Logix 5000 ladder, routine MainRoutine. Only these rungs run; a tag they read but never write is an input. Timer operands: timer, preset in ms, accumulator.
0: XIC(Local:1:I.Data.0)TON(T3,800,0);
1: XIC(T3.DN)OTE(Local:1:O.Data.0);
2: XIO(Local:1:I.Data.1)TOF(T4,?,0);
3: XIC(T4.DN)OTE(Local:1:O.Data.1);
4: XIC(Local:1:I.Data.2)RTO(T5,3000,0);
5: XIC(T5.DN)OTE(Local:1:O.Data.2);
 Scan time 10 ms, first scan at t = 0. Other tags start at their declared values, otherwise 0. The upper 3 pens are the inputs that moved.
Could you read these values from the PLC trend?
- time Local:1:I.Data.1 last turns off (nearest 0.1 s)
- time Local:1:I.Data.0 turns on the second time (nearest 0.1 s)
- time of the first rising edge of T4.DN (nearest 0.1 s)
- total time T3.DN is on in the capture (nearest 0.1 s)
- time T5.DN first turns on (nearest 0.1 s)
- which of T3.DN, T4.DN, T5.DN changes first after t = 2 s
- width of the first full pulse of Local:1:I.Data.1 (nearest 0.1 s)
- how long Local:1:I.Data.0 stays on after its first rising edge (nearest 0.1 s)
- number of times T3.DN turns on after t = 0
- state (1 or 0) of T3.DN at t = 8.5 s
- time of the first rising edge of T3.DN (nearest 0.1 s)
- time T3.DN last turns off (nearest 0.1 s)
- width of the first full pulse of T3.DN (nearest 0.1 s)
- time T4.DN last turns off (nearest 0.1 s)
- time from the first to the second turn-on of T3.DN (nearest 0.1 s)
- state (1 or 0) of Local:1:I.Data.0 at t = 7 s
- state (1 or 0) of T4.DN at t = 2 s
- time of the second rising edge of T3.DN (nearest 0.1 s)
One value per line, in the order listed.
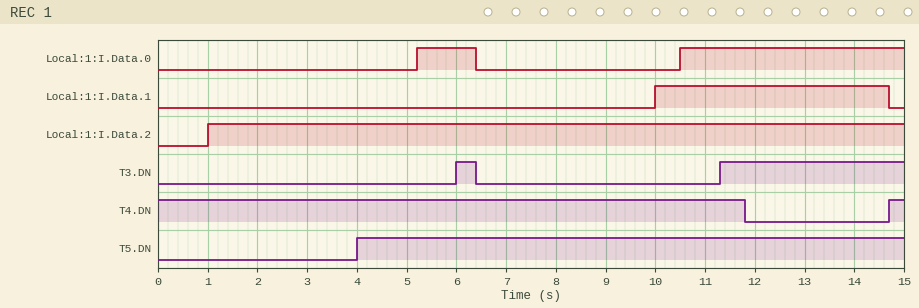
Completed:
14.7 s
10.5 s
14.7 s
4.1 s
4.0 s
T5.DN
4.7 s
1.2 s
2
0
6.0 s
6.4 s
0.4 s
11.8 s
5.3 s
0
1
11.3 s
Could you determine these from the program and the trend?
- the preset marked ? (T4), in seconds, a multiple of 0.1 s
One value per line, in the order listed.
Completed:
1.8 s
